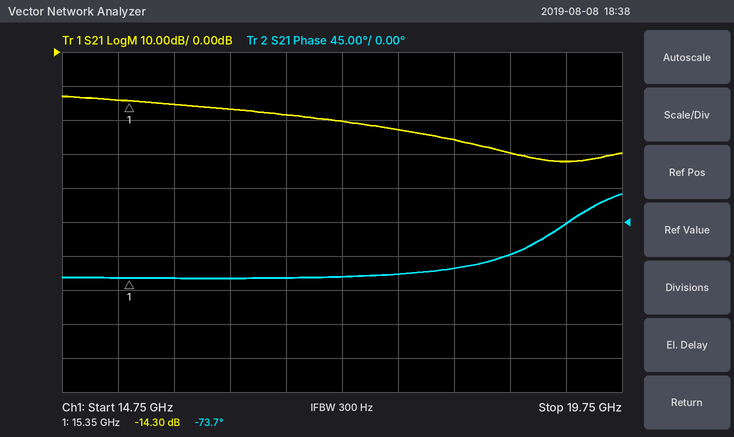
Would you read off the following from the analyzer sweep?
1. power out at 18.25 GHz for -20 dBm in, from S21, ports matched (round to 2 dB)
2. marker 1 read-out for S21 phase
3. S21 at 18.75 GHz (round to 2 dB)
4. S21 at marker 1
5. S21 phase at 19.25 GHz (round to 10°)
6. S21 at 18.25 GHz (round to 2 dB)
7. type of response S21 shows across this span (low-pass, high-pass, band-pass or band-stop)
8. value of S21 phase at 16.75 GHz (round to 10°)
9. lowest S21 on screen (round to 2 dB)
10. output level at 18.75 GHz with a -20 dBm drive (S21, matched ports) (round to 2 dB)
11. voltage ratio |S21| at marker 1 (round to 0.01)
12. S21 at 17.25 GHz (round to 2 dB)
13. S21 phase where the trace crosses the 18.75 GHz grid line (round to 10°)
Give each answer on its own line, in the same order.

-46 dBm
-73.7°
-30 dB
-14.30 dB
0°
-26 dB
low-pass
-70°
-32 dB
-50 dBm
0.19
-20 dB
-40°
